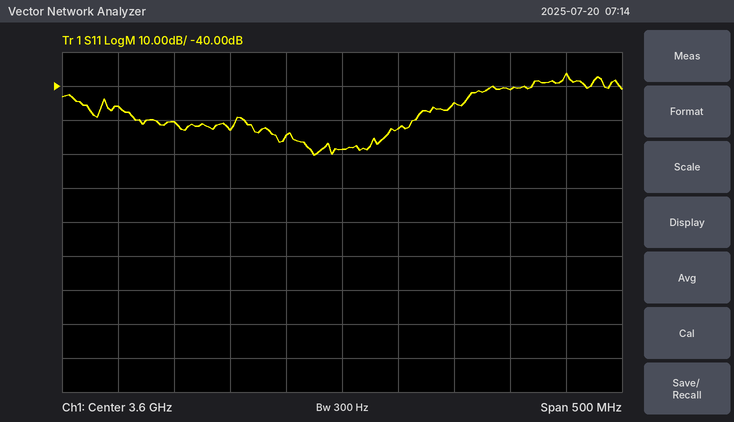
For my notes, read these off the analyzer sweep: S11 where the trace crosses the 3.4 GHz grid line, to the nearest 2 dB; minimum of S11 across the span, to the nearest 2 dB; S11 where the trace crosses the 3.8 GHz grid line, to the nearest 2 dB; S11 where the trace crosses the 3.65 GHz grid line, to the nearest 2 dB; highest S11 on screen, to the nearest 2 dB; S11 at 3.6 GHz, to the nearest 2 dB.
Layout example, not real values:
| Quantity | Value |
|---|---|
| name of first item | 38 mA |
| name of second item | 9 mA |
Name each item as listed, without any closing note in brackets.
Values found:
| Quantity | Value |
|---|---|
| S11 where the trace crosses the 3.4 GHz grid line, to the nearest 2 dB | -46 dB |
| minimum of S11 across the span, to the nearest 2 dB | -60 dB |
| S11 where the trace crosses the 3.8 GHz grid line, to the nearest 2 dB | -36 dB |
| S11 where the trace crosses the 3.65 GHz grid line, to the nearest 2 dB | -52 dB |
| highest S11 on screen, to the nearest 2 dB | -36 dB |
| S11 at 3.6 GHz, to the nearest 2 dB | -58 dB |
